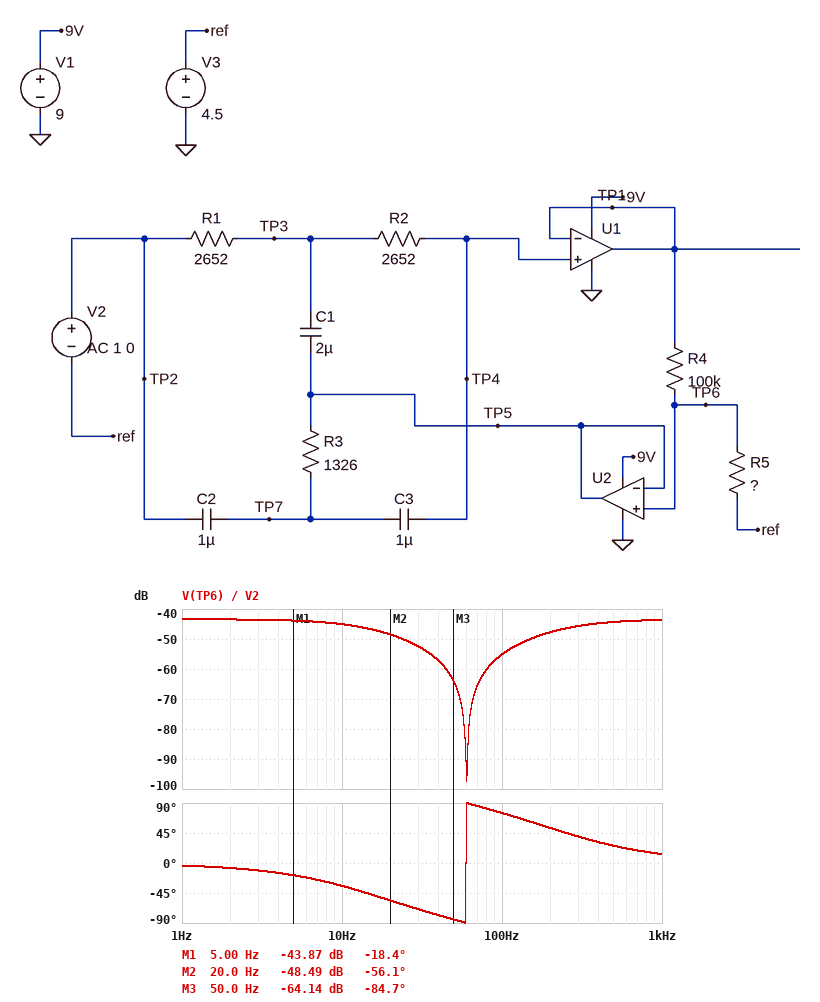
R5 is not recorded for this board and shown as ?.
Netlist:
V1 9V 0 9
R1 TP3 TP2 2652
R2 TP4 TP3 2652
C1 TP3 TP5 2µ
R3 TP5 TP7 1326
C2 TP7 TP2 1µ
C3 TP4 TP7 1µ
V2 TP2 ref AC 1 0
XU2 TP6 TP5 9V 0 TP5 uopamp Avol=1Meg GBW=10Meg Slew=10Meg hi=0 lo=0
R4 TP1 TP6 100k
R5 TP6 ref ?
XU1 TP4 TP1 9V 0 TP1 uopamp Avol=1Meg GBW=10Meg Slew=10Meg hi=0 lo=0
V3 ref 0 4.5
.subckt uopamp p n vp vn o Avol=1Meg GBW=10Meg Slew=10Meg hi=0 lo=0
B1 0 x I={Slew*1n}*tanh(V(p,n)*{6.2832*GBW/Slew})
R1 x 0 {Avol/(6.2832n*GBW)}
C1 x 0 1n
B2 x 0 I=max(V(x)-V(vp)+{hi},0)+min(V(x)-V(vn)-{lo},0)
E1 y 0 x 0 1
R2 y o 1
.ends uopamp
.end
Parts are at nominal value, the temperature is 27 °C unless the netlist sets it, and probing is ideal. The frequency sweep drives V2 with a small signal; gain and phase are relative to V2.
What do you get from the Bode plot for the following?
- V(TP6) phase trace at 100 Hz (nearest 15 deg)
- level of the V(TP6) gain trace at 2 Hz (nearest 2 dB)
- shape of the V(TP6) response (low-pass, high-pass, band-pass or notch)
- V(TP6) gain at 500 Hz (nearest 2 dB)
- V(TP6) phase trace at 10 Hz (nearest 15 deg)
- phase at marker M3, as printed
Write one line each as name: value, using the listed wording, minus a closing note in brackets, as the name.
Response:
V(TP6) phase trace at 100 Hz: 75 deg
level of the V(TP6) gain trace at 2 Hz: -44 dB
shape of the V(TP6) response: notch
V(TP6) gain at 500 Hz: -44 dB
V(TP6) phase trace at 10 Hz: -30 deg
phase at marker M3, as printed: -84.7 deg
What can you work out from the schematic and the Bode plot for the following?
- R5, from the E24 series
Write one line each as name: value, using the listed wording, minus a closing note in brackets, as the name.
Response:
R5, from the E24 series: 680 Ω
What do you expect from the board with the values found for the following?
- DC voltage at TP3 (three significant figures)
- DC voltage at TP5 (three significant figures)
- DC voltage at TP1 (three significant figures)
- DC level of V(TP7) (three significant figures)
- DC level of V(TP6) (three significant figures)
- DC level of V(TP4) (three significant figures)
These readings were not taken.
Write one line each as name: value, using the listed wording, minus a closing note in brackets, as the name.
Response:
DC voltage at TP3: 4.50 V
DC voltage at TP5: 4.50 V
DC voltage at TP1: 4.50 V
DC level of V(TP7): 4.50 V
DC level of V(TP6): 4.50 V
DC level of V(TP4): 4.50 V
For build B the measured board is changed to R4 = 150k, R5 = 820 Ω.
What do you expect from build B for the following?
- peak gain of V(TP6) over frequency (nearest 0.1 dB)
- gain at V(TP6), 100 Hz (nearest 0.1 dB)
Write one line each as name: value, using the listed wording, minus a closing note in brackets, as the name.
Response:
peak gain of V(TP6) over frequency: -45.3 dB
gain at V(TP6), 100 Hz: -57.0 dB
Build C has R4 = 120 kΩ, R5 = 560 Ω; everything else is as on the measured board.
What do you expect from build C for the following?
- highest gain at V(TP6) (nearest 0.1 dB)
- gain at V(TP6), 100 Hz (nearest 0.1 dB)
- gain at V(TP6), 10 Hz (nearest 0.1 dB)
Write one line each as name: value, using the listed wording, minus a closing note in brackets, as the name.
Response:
highest gain at V(TP6): -46.7 dB
gain at V(TP6), 100 Hz: -58.4 dB
gain at V(TP6), 10 Hz: -48.3 dB
